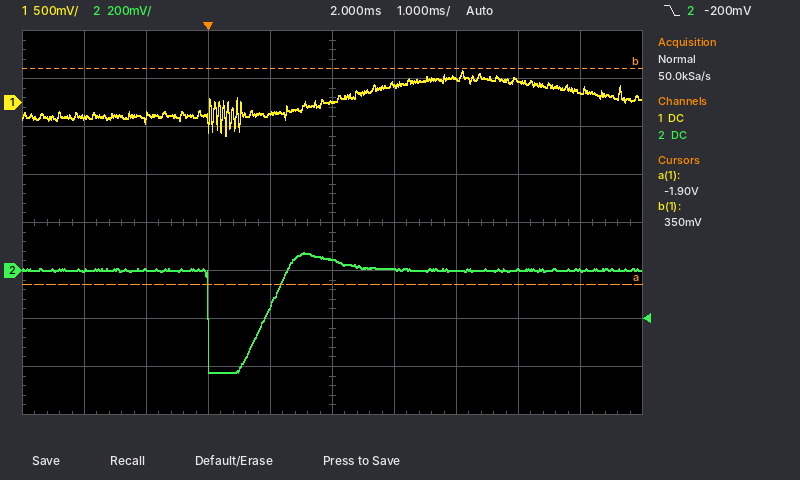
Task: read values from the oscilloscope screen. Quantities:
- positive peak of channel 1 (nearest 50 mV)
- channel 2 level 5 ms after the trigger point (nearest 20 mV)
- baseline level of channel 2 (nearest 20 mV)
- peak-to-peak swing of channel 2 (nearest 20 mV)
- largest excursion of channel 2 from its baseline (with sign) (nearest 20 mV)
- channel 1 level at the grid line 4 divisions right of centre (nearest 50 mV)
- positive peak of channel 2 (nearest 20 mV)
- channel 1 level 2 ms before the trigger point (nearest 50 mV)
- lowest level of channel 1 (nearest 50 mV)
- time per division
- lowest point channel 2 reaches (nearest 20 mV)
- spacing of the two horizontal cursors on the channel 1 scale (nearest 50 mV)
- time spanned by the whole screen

350 mV
0 mV
0 mV
500 mV
-420 mV
100 mV
80 mV
-150 mV
-350 mV
1 ms
-420 mV
2.25 V
10 ms
